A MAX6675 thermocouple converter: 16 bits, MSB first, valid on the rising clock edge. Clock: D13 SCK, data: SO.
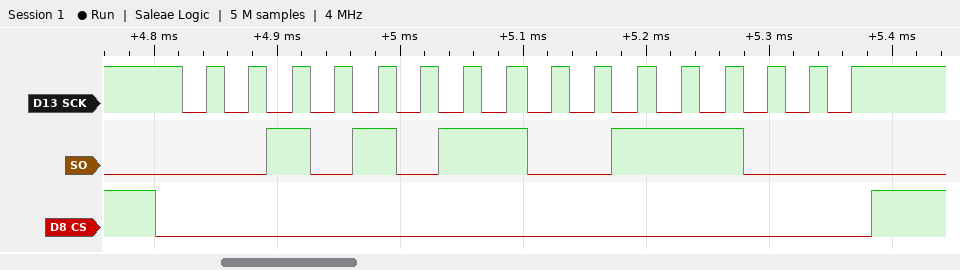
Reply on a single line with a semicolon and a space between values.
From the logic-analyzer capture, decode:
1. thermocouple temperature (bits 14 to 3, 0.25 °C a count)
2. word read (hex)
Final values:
345.75 °C; 0x2B38
